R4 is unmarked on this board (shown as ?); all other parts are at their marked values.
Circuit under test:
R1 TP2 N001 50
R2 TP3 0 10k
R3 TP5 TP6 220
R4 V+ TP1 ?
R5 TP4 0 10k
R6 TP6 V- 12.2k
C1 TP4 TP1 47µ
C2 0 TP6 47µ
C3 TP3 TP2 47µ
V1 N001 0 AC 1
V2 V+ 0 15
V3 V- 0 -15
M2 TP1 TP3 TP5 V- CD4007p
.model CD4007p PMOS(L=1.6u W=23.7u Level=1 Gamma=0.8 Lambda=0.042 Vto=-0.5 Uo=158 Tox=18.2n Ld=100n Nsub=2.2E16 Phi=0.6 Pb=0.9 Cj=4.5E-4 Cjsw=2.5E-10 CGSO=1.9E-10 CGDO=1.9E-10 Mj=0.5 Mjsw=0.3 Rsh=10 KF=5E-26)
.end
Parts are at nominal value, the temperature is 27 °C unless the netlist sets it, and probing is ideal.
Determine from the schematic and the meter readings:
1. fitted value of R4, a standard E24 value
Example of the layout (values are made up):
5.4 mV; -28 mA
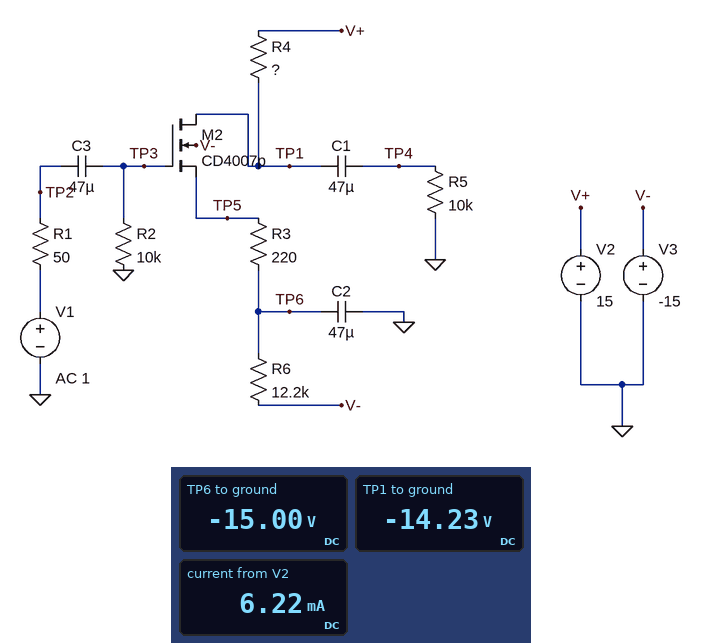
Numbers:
4.7 kΩ
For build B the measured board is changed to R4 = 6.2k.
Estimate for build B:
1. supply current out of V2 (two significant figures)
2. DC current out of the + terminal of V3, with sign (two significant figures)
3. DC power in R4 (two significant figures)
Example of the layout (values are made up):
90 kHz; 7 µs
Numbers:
4.7 mA; -4.7 mA; 140 mW
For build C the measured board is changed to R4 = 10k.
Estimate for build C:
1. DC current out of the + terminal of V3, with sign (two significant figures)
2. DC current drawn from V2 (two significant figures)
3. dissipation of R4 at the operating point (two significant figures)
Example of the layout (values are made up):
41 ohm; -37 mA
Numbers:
-2.9 mA; 2.9 mA; 86 mW
